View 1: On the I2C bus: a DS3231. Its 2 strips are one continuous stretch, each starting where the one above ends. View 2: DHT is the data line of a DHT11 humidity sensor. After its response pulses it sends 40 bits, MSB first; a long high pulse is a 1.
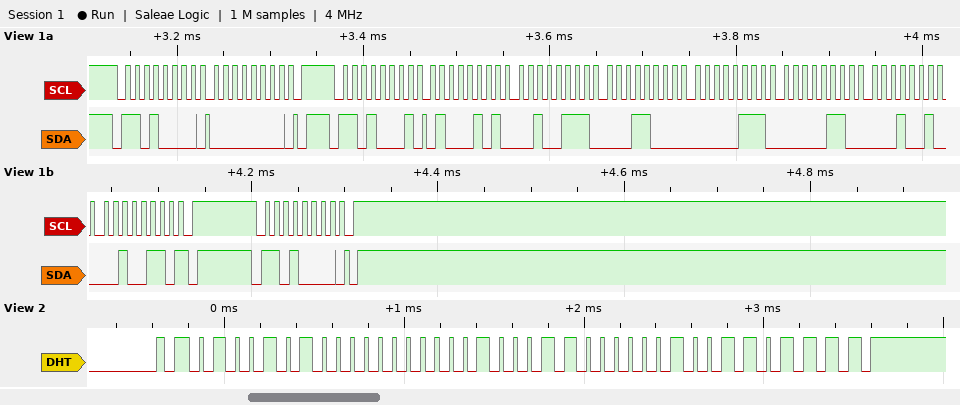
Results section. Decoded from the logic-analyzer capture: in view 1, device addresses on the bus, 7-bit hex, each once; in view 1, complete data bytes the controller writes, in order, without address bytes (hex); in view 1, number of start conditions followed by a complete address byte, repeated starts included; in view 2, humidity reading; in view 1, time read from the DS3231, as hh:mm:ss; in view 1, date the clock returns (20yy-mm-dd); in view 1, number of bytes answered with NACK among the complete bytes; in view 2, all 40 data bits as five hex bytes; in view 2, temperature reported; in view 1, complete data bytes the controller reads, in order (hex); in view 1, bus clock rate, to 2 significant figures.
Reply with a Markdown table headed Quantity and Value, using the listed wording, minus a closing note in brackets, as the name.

| Quantity | Value |
|---|---|
| in view 1, device addresses on the bus, 7-bit hex, each once | 0x68 |
| in view 1, complete data bytes the controller writes, in order, without address bytes | 00 |
| in view 1, number of start conditions followed by a complete address byte, repeated starts included | 3 |
| in view 2, humidity reading | 74 % |
| in view 1, time read from the DS3231, as hh:mm:ss | 18:27:45 |
| in view 1, date the clock returns | 2026-12-06 |
| in view 1, number of bytes answered with NACK among the complete bytes | 1 |
| in view 2, all 40 data bits as five hex bytes | 4A 00 23 02 6F |
| in view 2, temperature reported | 35.2 °C |
| in view 1, complete data bytes the controller reads, in order | 45 27 18 07 06 12 26 |
| in view 1, bus clock rate, to 2 significant figures | 100 kHz |
